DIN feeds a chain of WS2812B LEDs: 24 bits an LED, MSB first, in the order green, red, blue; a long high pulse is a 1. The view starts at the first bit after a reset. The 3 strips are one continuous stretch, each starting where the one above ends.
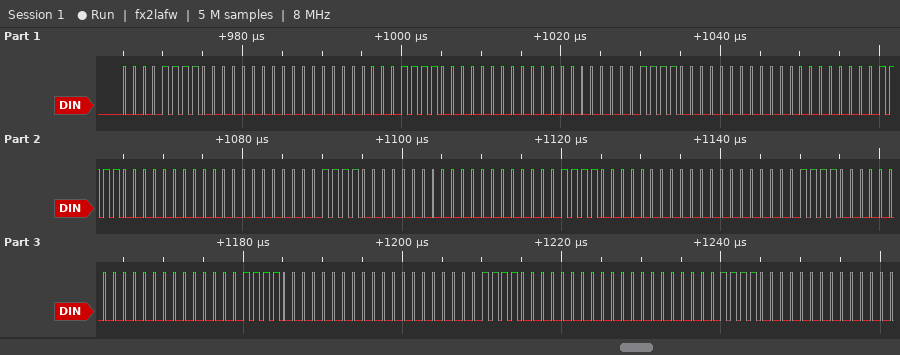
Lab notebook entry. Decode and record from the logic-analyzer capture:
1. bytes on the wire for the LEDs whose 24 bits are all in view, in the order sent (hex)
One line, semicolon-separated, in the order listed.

0F 00 00 0F 00 00 0F 00 00 0F 00 00 0F 00 00 0F 00 00 0F 00 00 0F 00 00 0F 00 00
